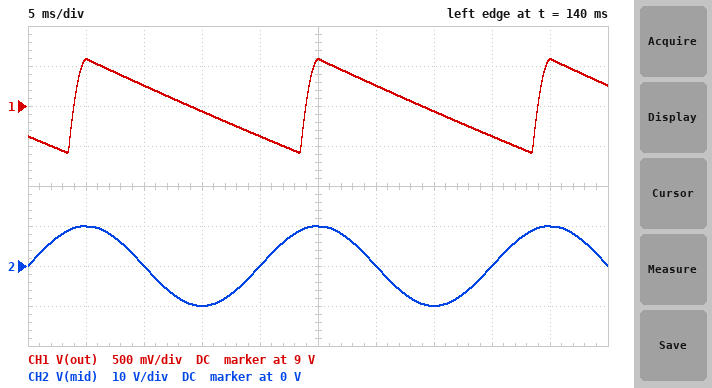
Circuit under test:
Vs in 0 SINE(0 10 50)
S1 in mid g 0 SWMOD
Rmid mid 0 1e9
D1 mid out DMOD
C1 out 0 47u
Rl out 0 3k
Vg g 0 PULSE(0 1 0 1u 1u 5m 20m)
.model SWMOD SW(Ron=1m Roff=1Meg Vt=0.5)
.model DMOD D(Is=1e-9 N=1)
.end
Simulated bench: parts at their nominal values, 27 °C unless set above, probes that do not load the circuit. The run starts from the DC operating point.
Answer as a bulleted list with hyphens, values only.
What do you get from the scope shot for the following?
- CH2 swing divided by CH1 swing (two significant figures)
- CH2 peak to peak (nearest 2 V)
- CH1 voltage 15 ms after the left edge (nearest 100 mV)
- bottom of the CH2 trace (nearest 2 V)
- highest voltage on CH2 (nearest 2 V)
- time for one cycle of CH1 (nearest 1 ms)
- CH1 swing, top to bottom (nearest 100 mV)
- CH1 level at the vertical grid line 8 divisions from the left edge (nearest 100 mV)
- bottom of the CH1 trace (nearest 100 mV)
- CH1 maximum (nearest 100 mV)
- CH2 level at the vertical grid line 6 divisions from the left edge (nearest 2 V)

- 17
- 20 V
- 8.9 V
- -10 V
- 10 V
- 20 ms
- 1.2 V
- 8.6 V
- 8.4 V
- 9.6 V
- 0 V
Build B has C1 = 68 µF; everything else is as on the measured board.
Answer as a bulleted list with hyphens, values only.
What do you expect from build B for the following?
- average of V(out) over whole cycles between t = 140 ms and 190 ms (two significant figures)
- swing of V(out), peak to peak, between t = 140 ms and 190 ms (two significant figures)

- 9.2 V
- 840 mV
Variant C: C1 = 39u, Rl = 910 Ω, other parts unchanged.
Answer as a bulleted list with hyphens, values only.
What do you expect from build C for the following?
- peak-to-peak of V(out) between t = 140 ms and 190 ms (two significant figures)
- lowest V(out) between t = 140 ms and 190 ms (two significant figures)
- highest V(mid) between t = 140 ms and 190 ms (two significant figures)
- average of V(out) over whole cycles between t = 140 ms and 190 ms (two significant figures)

- 3.7 V
- 5.9 V
- 10 V
- 7.7 V
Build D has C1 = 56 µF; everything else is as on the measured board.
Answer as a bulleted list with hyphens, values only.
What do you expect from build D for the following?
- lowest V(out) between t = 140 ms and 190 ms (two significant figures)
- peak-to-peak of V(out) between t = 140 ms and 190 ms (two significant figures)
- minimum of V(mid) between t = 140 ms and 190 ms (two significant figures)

- 8.6 V
- 1.0 V
- -10 V
